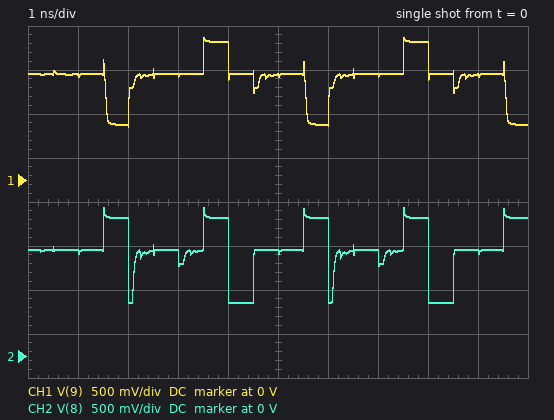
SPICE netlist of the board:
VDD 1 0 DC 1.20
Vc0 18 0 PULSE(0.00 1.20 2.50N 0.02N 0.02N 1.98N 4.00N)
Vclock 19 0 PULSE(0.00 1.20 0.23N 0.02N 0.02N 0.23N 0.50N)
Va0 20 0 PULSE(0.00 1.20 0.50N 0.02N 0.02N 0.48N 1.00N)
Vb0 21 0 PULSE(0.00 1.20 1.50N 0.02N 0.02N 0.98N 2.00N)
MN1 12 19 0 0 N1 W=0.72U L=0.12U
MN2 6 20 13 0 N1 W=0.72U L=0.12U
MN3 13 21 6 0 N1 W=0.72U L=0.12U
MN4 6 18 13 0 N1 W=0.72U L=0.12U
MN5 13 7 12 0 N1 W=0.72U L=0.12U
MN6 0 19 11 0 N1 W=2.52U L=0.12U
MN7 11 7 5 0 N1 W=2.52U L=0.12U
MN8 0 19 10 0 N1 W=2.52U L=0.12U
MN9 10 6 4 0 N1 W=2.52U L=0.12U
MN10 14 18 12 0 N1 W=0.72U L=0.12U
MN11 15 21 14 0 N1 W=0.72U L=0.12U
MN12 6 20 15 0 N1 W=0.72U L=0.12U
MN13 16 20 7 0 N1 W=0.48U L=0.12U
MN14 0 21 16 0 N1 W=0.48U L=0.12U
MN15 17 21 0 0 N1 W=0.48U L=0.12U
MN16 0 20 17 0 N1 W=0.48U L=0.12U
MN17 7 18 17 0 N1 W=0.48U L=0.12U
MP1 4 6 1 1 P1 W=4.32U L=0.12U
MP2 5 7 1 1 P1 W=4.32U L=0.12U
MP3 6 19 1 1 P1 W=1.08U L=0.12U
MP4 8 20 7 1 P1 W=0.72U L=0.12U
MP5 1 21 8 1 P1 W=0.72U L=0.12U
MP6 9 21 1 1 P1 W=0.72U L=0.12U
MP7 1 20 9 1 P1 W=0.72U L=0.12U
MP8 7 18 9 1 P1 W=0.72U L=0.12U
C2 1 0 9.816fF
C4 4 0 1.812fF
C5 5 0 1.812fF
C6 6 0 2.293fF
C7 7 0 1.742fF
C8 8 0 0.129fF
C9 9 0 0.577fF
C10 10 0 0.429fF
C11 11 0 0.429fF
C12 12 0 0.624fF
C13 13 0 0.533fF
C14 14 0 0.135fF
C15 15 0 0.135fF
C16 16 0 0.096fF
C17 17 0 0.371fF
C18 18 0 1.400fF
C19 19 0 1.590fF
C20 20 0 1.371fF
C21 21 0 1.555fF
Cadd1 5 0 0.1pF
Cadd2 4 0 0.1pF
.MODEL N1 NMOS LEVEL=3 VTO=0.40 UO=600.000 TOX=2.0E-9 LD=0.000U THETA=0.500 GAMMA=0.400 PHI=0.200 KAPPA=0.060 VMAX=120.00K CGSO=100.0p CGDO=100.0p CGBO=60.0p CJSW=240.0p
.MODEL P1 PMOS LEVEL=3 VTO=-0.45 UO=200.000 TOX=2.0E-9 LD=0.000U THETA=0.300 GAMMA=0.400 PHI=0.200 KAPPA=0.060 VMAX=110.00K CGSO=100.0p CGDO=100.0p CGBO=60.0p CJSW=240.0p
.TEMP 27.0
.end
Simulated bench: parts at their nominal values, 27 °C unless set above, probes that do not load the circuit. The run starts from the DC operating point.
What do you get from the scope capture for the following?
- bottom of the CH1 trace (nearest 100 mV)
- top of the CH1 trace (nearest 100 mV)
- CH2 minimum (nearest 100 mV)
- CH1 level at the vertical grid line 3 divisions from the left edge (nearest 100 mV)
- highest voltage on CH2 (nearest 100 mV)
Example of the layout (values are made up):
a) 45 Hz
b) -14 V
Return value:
a) 600 mV
b) 1.6 V
c) 600 mV
d) 1.2 V
e) 1.7 V
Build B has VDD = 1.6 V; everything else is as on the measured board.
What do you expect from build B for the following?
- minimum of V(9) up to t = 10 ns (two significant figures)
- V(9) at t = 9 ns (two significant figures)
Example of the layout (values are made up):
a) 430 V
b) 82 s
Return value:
a) 690 mV
b) 1.6 V
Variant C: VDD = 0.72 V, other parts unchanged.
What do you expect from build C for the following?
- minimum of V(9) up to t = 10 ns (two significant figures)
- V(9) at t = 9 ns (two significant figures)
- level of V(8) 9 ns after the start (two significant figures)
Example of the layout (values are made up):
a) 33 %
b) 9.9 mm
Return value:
a) 480 mV
b) 710 mV
c) 720 mV
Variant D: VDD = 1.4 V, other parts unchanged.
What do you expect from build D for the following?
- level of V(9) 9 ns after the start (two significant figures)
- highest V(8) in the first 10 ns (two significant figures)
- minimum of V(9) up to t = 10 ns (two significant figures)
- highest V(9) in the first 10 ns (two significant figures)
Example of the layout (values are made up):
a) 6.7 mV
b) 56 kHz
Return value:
a) 1.4 V
b) 1.7 V
c) 650 mV
d) 1.7 V
